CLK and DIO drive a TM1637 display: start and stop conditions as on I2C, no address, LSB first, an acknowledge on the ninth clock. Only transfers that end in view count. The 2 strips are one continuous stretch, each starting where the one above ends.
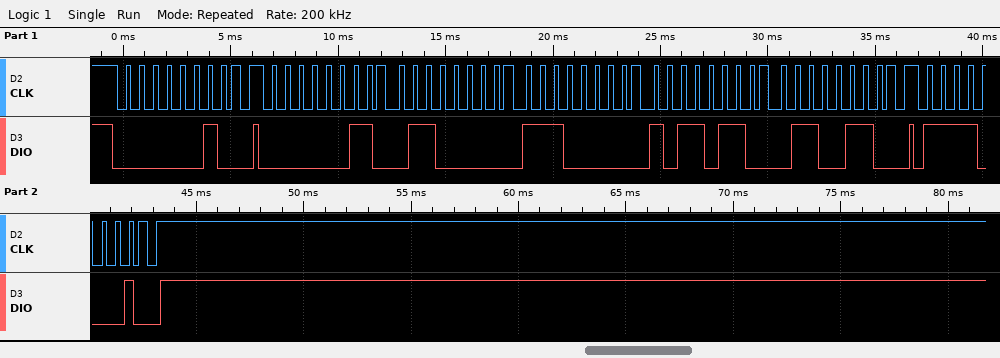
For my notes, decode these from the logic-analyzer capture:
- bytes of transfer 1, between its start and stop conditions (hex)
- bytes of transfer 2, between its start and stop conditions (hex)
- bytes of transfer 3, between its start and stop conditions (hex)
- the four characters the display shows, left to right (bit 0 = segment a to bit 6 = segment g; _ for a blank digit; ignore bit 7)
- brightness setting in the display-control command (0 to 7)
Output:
40
C0 06 07 6D 66
8F
1754
7
